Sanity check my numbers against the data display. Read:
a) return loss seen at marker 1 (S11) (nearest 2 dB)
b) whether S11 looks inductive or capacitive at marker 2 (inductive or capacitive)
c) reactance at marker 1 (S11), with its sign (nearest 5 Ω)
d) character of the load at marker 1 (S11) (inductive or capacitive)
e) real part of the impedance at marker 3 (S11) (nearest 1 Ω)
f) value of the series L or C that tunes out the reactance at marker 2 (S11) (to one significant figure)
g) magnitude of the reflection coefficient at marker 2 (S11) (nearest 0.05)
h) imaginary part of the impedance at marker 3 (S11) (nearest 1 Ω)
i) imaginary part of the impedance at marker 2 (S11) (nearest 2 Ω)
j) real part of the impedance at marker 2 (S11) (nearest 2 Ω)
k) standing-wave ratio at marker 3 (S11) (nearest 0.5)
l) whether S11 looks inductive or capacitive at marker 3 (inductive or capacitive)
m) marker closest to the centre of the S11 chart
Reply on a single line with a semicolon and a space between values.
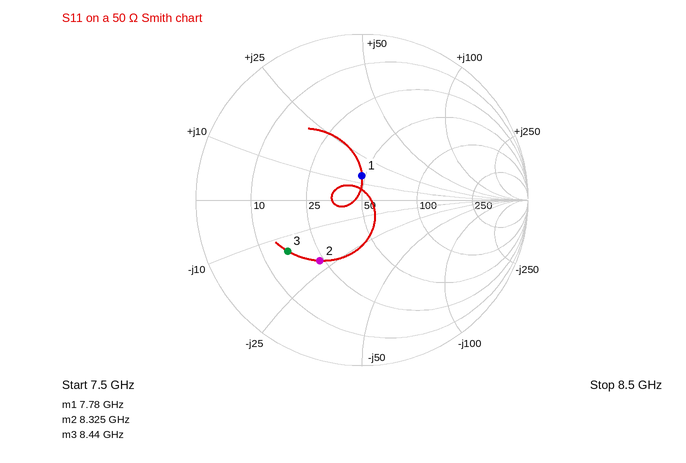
16 dB; capacitive; +15 Ω; inductive; 16 Ω; 400 pH; 0.45; -14 Ω; -22 Ω; 24 Ω; 3.5; capacitive; marker 1
